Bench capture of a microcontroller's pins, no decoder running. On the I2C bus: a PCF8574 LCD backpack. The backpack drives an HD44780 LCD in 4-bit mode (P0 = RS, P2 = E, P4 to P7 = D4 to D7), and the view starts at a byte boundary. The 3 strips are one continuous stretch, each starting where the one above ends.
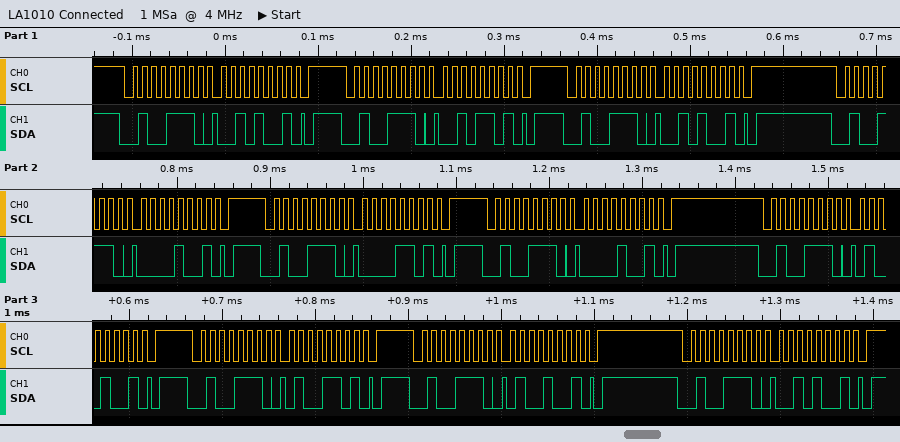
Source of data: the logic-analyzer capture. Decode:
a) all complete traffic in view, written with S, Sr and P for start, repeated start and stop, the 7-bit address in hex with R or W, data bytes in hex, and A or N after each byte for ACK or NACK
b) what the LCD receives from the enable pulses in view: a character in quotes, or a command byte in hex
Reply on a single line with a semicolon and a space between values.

S 27W A 29 A P S 27W A 2D A P S 27W A 29 A P S 27W A 09 A P S 27W A 0D A P S 27W A 09 A P S 27W A 49 A P S 27W A 4D A P S 27W A 49 A P S 27W A 29 A P; ' '
